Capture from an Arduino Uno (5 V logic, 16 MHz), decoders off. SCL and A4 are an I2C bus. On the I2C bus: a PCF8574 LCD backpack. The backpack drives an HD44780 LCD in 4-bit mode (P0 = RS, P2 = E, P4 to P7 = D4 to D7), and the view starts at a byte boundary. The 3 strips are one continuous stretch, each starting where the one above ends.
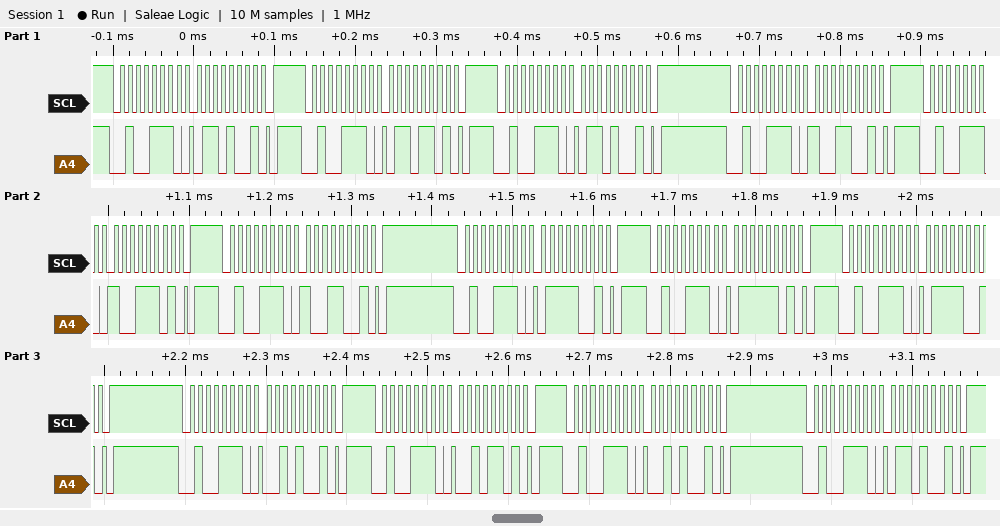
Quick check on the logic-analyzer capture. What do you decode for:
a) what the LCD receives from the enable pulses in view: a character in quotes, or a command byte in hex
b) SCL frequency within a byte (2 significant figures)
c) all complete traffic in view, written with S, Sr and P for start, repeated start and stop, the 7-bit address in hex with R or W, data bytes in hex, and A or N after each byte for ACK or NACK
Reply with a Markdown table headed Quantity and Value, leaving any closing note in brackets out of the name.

| Quantity | Value |
|---|---|
| what the LCD receives from the enable pulses in view: a character in quotes, or a command byte in hex | 'i' 'r' |
| SCL frequency within a byte | 100 kHz |
| all complete traffic in view, written with S, Sr and P for start, repeated start and stop, the 7-bit address in hex with R or W, data bytes in hex, and A or N after each byte for ACK or NACK | S 27W A 69 A P S 27W A 6D A P S 27W A 69 A P S 27W A 99 A P S 27W A 9D A P S 27W A 99 A P S 27W A 79 A P S 27W A 7D A P S 27W A 79 A P S 27W A 29 A P S 27W A 2D A P S 27W A 29 A P S 27W A 69 A P |
